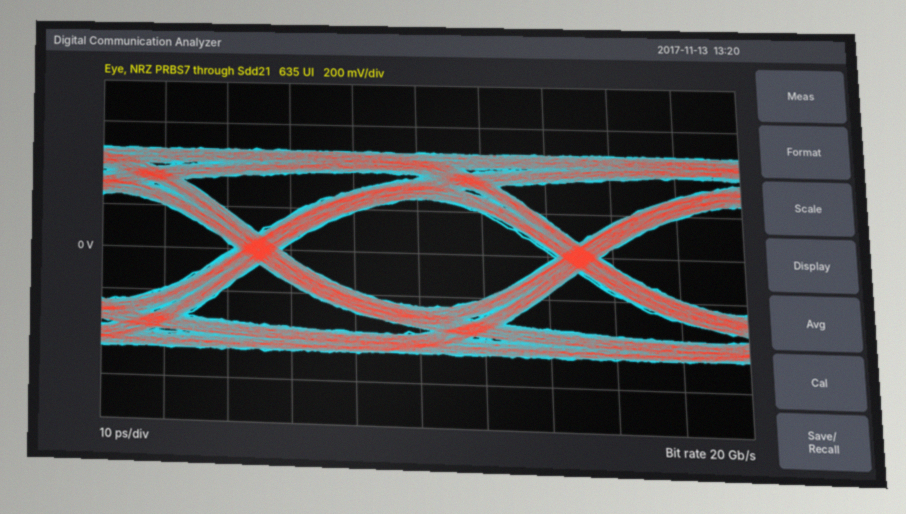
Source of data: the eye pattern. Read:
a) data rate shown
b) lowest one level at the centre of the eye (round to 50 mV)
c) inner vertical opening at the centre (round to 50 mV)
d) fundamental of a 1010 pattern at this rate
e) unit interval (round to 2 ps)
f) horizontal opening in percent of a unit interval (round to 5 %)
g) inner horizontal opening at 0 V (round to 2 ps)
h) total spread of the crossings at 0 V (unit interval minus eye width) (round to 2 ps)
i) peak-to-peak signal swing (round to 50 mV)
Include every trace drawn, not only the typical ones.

20 Gb/s
250 mV
500 mV
10 GHz
50 ps
85 %
42 ps
8 ps
950 mV
